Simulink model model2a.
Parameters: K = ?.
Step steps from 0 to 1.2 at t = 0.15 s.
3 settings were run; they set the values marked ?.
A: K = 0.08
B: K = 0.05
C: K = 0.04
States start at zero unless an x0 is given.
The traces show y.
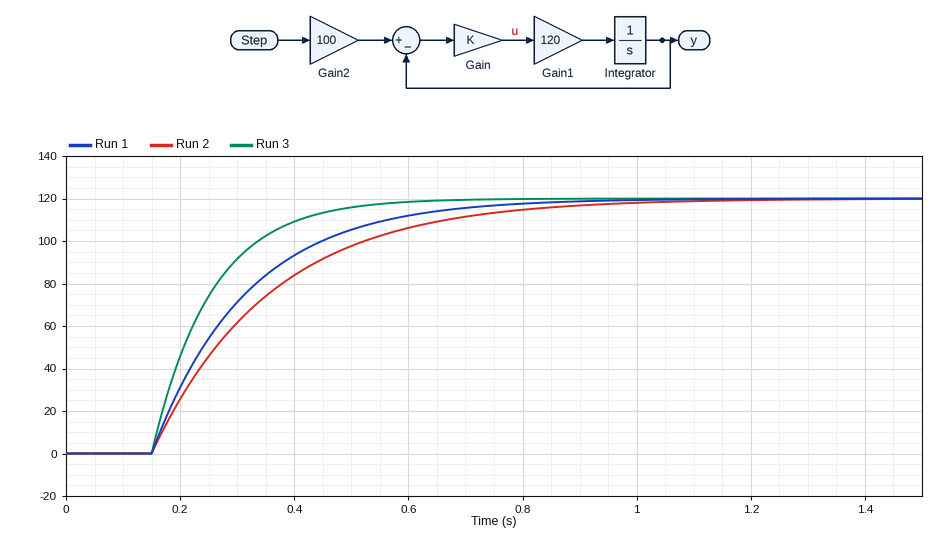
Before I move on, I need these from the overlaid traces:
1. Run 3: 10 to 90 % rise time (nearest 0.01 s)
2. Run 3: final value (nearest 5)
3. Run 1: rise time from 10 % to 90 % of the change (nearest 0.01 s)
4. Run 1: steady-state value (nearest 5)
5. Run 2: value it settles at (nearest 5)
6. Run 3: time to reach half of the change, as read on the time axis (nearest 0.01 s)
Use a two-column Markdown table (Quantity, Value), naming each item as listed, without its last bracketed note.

| Quantity | Value |
|---|---|
| Run 3: 10 to 90 % rise time | 0.23 s |
| Run 3: final value | 120 |
| Run 1: rise time from 10 % to 90 % of the change | 0.37 s |
| Run 1: steady-state value | 120 |
| Run 2: value it settles at | 120 |
| Run 3: time to reach half of the change, as read on the time axis | 0.22 s |
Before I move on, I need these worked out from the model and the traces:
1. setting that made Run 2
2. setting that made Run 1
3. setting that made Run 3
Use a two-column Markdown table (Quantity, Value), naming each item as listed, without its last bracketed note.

| Quantity | Value |
|---|---|
| setting that made Run 2 | C |
| setting that made Run 1 | B |
| setting that made Run 3 | A |
